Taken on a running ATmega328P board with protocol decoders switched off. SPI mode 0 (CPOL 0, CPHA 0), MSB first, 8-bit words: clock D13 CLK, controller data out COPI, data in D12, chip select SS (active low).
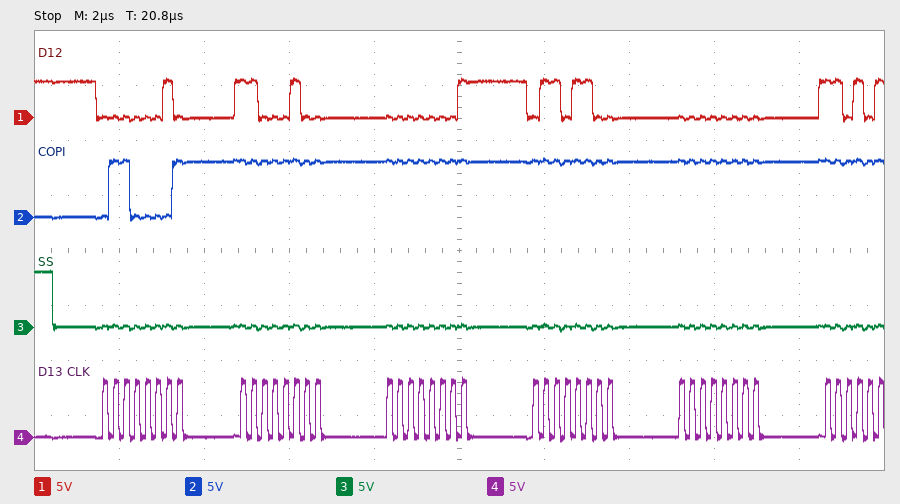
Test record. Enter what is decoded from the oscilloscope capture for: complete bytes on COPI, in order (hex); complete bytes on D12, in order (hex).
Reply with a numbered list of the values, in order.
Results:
1. 61 FF FF FF FF
2. 02 C4 01 6C 00
